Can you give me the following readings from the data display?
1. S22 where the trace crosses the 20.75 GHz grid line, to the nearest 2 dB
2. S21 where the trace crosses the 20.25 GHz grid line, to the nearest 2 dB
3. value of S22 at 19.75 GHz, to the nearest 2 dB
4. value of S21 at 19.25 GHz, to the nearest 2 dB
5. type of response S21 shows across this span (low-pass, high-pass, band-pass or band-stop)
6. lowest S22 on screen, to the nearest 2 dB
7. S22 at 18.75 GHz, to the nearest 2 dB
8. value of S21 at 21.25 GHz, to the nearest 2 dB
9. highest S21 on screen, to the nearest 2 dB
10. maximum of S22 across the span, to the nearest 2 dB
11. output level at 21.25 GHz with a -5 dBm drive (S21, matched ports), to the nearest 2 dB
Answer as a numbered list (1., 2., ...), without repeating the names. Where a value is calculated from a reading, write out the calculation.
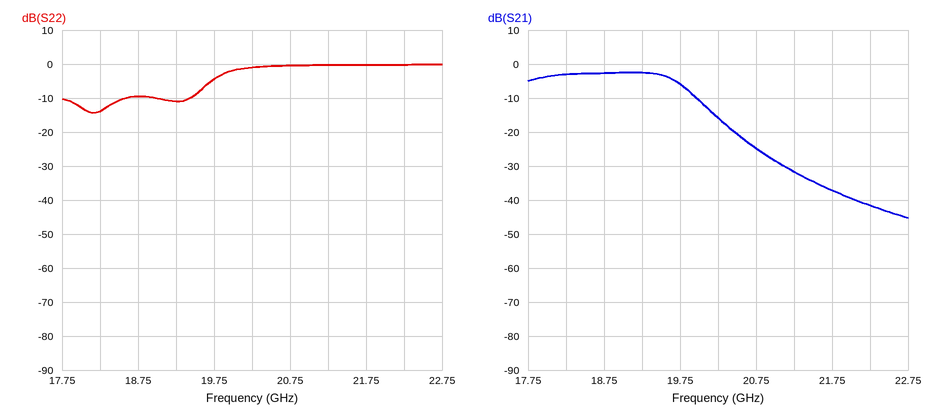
1. 0 dB
2. -16 dB
3. -4 dB
4. -2 dB
5. low-pass
6. -14 dB
7. -10 dB
8. -32 dB
9. -2 dB
10. 0 dB
11. -5 dBm + (-32 dB) = -36 dBm
